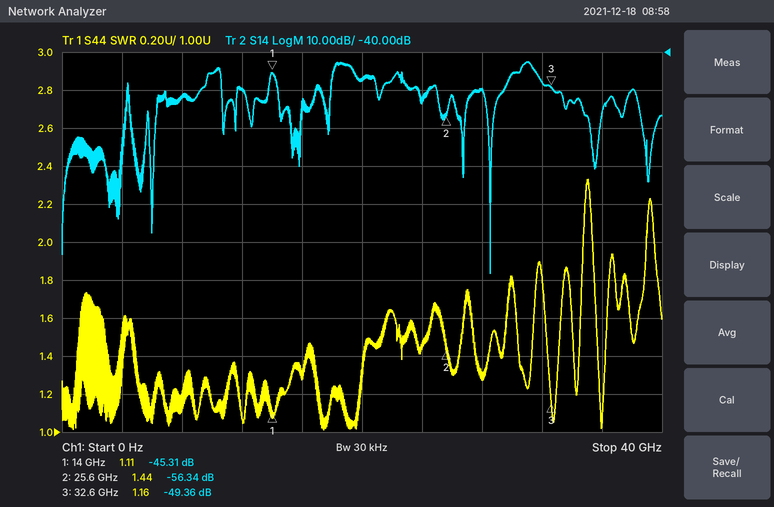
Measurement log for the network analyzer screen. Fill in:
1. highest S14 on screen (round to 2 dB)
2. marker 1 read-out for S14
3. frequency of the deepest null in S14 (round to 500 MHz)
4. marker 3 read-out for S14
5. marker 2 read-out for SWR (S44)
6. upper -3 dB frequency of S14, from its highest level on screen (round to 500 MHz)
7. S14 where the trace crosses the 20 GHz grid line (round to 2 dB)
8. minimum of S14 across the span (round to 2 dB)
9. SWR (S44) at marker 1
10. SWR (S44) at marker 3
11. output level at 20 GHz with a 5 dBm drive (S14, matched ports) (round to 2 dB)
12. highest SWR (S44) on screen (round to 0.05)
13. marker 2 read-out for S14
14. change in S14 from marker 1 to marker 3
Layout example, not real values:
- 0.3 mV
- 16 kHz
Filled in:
- -42 dB
- -45.31 dB
- 28.5 GHz
- -49.36 dB
- 1.44
- 31.5 GHz
- -48 dB
- -98 dB
- 1.11
- 1.16
- -42 dBm
- 2.35
- -56.34 dB
- -4.05 dB
